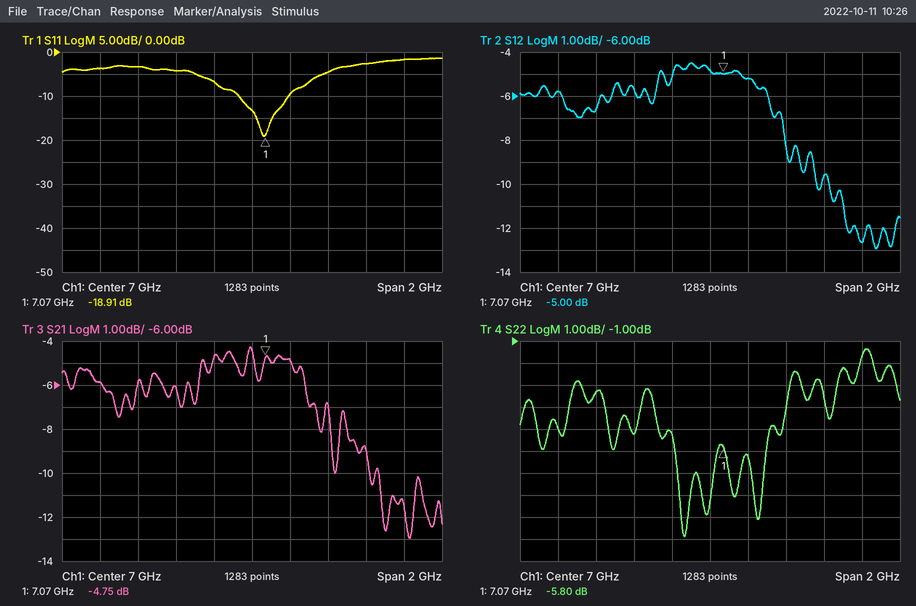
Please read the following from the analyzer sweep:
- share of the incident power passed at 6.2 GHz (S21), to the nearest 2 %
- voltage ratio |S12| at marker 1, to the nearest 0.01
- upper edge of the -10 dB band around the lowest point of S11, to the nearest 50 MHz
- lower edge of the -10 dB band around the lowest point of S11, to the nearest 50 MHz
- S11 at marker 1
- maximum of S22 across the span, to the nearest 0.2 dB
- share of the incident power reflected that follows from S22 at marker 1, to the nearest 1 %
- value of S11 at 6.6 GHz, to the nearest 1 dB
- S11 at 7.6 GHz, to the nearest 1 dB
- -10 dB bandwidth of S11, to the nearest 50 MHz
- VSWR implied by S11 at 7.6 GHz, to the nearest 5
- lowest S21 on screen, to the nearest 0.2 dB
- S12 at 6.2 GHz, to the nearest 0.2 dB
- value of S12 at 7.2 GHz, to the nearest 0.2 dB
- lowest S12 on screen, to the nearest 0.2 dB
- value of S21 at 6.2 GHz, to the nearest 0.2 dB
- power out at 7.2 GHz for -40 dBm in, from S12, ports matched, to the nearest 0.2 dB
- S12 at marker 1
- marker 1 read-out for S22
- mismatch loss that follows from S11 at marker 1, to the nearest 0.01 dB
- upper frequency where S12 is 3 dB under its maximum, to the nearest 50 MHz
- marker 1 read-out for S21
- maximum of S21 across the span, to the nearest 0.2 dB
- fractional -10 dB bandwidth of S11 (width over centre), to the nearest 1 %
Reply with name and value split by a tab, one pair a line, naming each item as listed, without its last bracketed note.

share of the incident power passed at 6.2 GHz (S21), to the nearest 2 %	26 %
voltage ratio |S12| at marker 1, to the nearest 0.01	0.56
upper edge of the -10 dB band around the lowest point of S11, to the nearest 50 MHz	7.20 GHz
lower edge of the -10 dB band around the lowest point of S11, to the nearest 50 MHz	6.95 GHz
S11 at marker 1	-18.91 dB
maximum of S22 across the span, to the nearest 0.2 dB	-1.4 dB
share of the incident power reflected that follows from S22 at marker 1, to the nearest 1 %	26 %
value of S11 at 6.6 GHz, to the nearest 1 dB	-4 dB
S11 at 7.6 GHz, to the nearest 1 dB	-3 dB
-10 dB bandwidth of S11, to the nearest 50 MHz	250 MHz
VSWR implied by S11 at 7.6 GHz, to the nearest 5	5
lowest S21 on screen, to the nearest 0.2 dB	-13.0 dB
S12 at 6.2 GHz, to the nearest 0.2 dB	-5.8 dB
value of S12 at 7.2 GHz, to the nearest 0.2 dB	-5.2 dB
lowest S12 on screen, to the nearest 0.2 dB	-13.0 dB
value of S21 at 6.2 GHz, to the nearest 0.2 dB	-5.8 dB
power out at 7.2 GHz for -40 dBm in, from S12, ports matched, to the nearest 0.2 dB	-45.2 dBm
S12 at marker 1	-5.00 dB
marker 1 read-out for S22	-5.80 dB
mismatch loss that follows from S11 at marker 1, to the nearest 0.01 dB	0.06 dB
upper frequency where S12 is 3 dB under its maximum, to the nearest 50 MHz	7.40 GHz
marker 1 read-out for S21	-4.75 dB
maximum of S21 across the span, to the nearest 0.2 dB	-4.2 dB
fractional -10 dB bandwidth of S11 (width over centre), to the nearest 1 %	4 %
